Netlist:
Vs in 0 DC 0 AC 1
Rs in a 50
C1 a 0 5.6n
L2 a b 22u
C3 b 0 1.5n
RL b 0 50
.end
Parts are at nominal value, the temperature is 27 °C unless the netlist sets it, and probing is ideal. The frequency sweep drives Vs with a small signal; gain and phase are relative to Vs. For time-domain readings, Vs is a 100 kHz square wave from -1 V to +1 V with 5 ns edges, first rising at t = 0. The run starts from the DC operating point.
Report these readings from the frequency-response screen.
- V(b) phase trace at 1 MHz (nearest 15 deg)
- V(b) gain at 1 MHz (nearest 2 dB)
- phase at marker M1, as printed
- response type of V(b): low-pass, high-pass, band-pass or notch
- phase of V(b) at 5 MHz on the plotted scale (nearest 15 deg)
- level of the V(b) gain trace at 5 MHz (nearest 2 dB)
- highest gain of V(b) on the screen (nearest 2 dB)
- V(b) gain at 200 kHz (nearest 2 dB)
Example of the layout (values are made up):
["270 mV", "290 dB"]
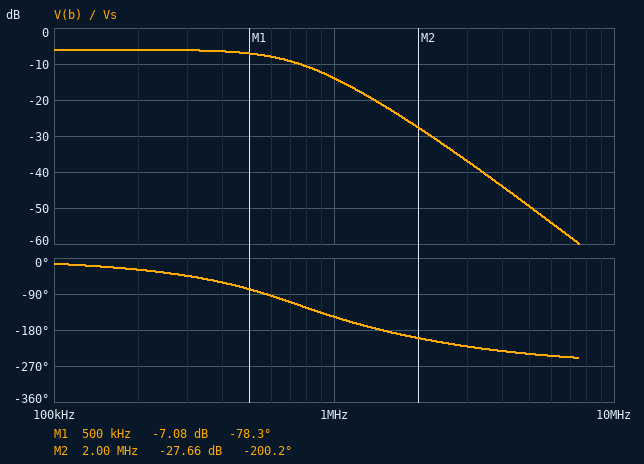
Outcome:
["-150 deg", "-14 dB", "-78.3 deg", "low-pass", "-240 deg", "-50 dB", "-6 dB", "-6 dB"]
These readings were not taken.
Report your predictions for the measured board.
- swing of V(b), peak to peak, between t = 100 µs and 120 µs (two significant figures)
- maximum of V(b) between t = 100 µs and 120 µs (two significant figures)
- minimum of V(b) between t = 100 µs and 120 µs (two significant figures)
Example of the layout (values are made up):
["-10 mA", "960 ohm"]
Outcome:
["1.1 V", "550 mV", "-550 mV"]
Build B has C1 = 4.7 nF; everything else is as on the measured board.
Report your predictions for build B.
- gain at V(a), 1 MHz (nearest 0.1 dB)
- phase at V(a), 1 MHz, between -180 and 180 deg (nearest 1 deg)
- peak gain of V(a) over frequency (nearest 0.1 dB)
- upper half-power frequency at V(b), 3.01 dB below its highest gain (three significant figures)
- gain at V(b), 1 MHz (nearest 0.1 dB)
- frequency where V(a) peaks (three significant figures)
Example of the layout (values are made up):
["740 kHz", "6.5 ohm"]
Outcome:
["-4.0 dB", "-44 deg", "-2.8 dB", "730 kHz", "-12.8 dB", "663 kHz"]
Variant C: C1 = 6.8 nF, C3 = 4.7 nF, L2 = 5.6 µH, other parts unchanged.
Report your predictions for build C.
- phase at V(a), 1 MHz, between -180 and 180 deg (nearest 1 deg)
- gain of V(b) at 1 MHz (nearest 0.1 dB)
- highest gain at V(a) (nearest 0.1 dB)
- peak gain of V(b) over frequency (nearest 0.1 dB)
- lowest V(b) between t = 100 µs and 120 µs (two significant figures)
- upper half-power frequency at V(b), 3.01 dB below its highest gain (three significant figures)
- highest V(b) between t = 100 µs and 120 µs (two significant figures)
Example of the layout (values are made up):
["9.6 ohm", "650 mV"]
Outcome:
["-11 deg", "-6.7 dB", "-6.0 dB", "-6.0 dB", "-530 mV", "1.38 MHz", "530 mV"]
